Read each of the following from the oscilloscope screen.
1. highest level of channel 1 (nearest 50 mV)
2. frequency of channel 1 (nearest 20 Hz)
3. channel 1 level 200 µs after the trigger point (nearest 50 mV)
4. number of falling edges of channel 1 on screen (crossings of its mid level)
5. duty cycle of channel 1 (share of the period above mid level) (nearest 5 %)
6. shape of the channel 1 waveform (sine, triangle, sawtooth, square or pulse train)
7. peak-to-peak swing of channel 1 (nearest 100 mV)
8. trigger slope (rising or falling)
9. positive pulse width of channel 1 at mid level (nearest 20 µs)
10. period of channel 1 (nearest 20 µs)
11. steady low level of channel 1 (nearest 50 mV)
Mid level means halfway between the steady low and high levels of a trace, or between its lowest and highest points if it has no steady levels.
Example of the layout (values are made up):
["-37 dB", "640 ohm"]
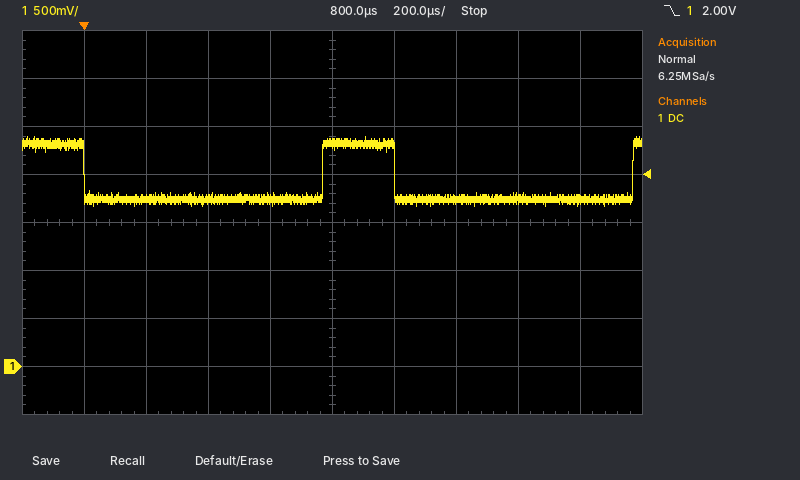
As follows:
["2.40 V", "1.00 kHz", "1.75 V", "2", "25 %", "pulse train", "700 mV", "falling", "240 µs", "1.00 ms", "1.75 V"]
